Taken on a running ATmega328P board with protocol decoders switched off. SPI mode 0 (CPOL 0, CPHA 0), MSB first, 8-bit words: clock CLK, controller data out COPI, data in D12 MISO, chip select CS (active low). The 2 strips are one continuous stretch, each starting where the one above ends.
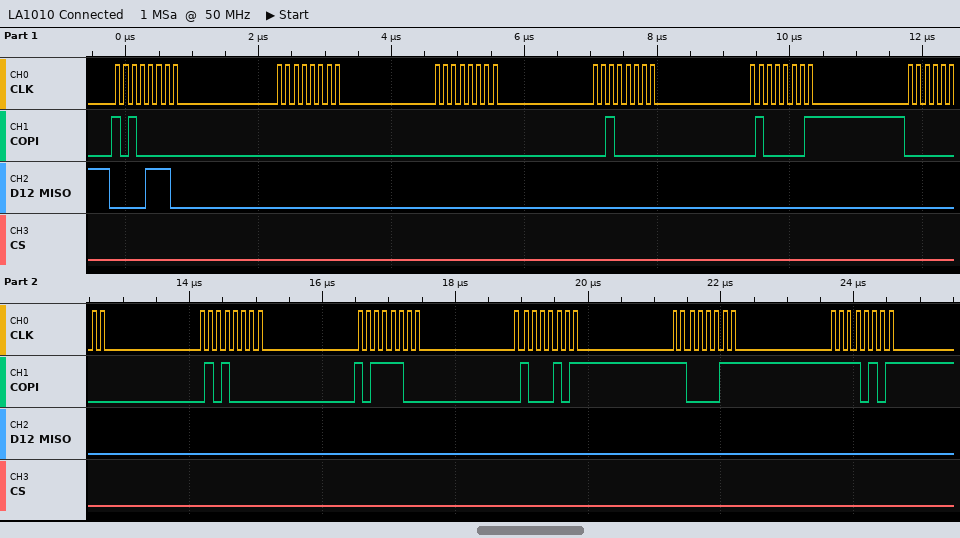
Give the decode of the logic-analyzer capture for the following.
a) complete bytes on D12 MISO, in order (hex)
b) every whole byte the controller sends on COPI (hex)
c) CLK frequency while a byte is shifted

0E 00 00 00 00 00 00 00 00 00 00
A0 00 00 20 41 00 50 BC 45 C3 F5
8 MHz
